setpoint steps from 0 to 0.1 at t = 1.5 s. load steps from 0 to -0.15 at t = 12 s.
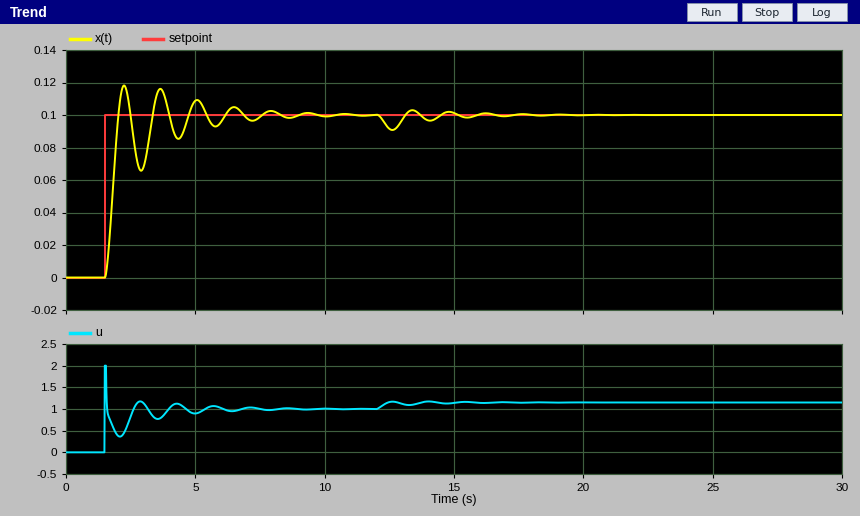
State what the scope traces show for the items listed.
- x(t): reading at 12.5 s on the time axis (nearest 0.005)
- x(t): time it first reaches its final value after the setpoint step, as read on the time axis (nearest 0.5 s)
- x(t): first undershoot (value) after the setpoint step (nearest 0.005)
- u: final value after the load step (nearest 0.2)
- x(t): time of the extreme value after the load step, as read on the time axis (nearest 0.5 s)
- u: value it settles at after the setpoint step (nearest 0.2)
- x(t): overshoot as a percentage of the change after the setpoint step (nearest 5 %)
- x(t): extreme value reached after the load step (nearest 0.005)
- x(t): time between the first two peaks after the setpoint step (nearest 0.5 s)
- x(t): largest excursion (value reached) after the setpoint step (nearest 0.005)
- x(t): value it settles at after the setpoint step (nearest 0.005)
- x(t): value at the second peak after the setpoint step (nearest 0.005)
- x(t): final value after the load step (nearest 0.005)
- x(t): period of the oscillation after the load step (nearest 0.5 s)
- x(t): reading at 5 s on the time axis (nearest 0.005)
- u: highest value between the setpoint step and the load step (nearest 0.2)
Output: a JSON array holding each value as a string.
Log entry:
["0.090", "2.0 s", "0.065", "1.2", "12.5 s", "1.0", "20 %", "0.090", "1.5 s", "0.120", "0.100", "0.115", "0.100", "1.5 s", "0.110", "2.0"]
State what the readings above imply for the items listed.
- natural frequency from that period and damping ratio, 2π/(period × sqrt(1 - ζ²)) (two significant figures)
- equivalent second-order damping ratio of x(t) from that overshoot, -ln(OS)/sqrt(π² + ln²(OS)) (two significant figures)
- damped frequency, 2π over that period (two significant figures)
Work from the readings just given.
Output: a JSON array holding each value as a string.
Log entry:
["4.7 rad/s", "0.46", "4.2 rad/s"]
